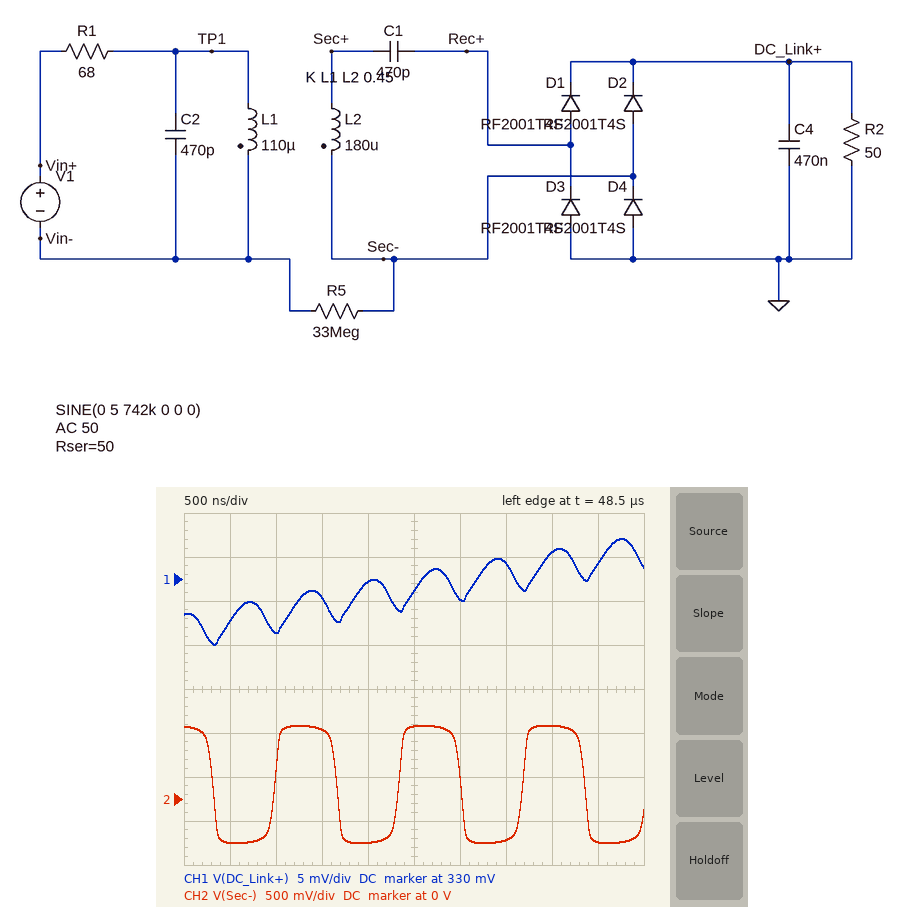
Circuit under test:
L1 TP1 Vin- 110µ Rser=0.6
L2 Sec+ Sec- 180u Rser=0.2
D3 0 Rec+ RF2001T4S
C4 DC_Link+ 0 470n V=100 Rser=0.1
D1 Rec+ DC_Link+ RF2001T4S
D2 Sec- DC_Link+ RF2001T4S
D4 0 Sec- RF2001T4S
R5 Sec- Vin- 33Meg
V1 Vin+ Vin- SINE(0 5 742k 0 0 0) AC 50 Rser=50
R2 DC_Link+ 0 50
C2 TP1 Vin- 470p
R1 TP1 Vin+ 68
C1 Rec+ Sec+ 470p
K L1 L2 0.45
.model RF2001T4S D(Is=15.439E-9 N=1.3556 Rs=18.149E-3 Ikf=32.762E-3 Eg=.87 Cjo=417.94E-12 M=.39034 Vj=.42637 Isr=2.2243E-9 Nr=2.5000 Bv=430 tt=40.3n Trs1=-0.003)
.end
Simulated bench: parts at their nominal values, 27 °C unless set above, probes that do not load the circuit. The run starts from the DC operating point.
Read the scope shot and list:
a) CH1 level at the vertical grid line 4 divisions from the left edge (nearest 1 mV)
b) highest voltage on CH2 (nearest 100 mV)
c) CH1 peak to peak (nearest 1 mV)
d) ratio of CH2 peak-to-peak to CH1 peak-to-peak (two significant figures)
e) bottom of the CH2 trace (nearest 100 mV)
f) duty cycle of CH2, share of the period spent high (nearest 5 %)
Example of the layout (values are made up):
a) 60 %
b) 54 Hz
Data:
a) 330 mV
b) 800 mV
c) 12 mV
d) 110
e) -500 mV
f) 50 %
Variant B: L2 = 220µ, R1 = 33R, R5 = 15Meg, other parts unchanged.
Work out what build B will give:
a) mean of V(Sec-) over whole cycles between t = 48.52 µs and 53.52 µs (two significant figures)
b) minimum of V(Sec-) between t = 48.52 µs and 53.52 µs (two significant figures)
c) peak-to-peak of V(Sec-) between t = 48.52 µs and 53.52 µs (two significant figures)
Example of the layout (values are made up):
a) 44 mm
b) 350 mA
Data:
a) 110 mV
b) -490 mV
c) 1.2 V
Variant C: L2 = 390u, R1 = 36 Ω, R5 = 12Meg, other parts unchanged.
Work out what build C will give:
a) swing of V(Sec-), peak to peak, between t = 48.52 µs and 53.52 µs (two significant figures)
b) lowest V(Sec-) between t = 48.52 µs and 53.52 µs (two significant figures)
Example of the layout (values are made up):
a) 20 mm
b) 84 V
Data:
a) 1.0 V
b) -450 mV
